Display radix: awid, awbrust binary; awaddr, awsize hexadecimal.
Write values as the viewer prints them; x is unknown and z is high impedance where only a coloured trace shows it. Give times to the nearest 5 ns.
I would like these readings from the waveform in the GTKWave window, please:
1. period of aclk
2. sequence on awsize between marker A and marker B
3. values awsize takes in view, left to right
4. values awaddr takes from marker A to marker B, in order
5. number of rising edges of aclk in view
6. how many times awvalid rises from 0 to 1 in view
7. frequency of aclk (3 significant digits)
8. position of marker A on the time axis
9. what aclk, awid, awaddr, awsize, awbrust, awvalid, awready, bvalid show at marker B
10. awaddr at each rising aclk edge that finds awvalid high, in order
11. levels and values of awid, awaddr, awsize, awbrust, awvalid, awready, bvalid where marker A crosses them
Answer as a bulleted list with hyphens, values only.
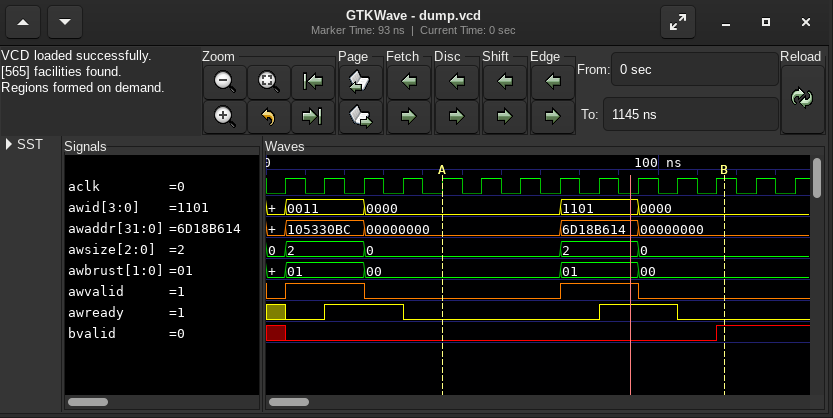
- 10 ns
- 0, 2, 0
- 0, 2, 0, 2, 0
- 00000000, 6D18B614, 00000000
- 14
- 2
- 100 MHz
- 45 ns
- aclk=1, awid=0000, awaddr=00000000, awsize=0, awbrust=00, awvalid=0, awready=0, bvalid=1
- 105330BC, 105330BC, 6D18B614, 6D18B614
- awid=0000, awaddr=00000000, awsize=0, awbrust=00, awvalid=0, awready=0, bvalid=0
